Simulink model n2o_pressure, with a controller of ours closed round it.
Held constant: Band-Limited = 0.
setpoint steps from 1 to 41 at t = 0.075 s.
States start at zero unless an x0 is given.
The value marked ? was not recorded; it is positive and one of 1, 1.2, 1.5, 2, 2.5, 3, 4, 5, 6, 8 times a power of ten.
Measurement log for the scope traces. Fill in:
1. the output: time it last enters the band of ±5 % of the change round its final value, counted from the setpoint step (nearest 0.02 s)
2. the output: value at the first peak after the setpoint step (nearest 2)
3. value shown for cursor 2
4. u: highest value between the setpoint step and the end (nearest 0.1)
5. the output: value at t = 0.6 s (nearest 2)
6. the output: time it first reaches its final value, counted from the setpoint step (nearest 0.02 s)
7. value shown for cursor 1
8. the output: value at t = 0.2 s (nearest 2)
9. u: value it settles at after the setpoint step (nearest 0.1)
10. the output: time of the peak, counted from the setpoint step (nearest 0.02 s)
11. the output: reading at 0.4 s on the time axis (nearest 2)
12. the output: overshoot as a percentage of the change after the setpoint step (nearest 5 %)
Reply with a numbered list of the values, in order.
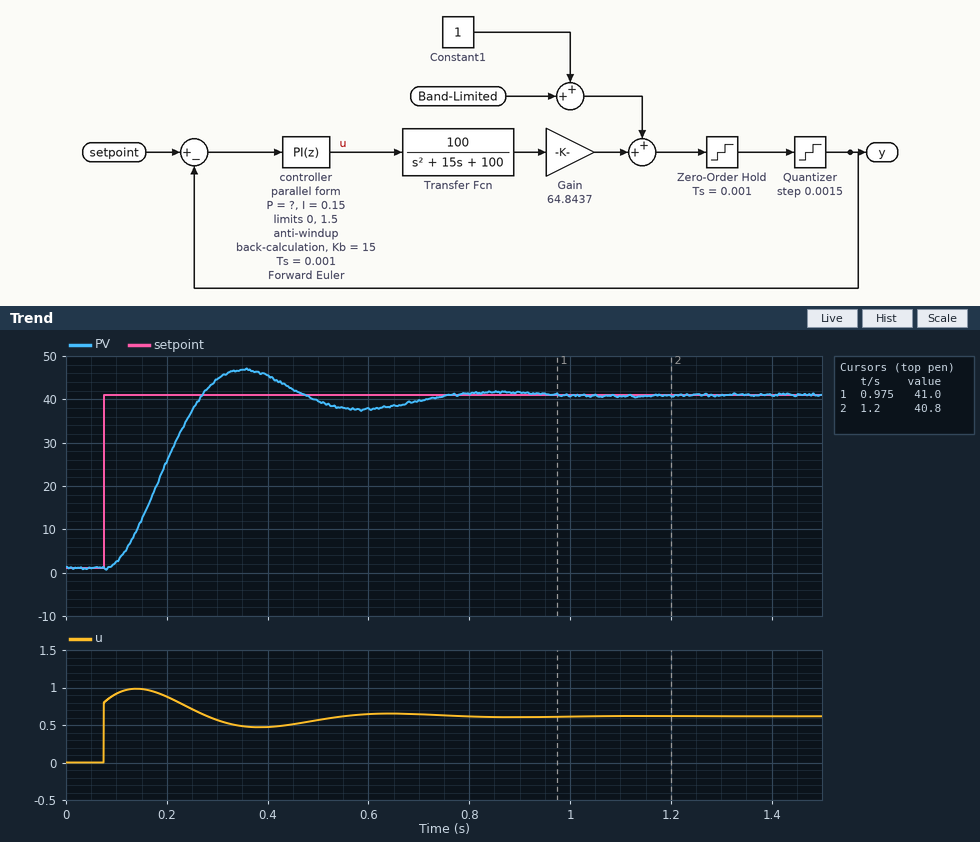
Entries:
1. 0.60 s
2. 46
3. 40.8
4. 1.0
5. 38
6. 0.20 s
7. 41.0
8. 26
9. 0.6
10. 0.28 s
11. 46
12. 15 %
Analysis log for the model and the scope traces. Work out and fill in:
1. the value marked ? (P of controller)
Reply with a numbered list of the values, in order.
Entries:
1. 0.02
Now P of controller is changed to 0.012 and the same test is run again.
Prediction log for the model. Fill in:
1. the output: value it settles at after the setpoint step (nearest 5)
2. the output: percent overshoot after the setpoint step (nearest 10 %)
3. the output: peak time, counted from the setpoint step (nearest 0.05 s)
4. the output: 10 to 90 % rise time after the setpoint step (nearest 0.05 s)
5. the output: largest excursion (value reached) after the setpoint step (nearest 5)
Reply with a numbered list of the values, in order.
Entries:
1. 40
2. 20 %
3. 0.35 s
4. 0.15 s
5. 50
